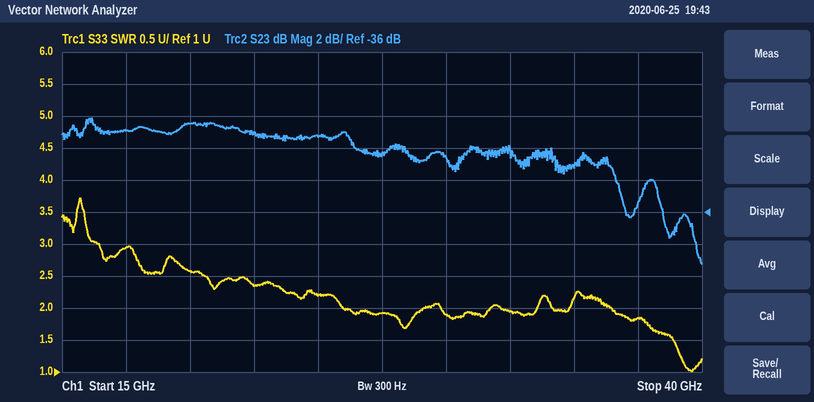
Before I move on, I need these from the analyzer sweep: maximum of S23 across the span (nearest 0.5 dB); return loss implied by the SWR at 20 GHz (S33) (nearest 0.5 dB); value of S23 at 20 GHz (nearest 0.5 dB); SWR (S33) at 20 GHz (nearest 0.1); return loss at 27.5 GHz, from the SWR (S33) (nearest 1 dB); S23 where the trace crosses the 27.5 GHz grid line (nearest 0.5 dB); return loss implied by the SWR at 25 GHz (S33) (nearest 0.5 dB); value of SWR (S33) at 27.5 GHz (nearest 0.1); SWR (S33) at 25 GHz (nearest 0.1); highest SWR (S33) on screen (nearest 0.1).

-30.0 dB
7.0 dB
-30.5 dB
2.6
10 dB
-32.5 dB
8.5 dB
1.9
2.2
3.7
